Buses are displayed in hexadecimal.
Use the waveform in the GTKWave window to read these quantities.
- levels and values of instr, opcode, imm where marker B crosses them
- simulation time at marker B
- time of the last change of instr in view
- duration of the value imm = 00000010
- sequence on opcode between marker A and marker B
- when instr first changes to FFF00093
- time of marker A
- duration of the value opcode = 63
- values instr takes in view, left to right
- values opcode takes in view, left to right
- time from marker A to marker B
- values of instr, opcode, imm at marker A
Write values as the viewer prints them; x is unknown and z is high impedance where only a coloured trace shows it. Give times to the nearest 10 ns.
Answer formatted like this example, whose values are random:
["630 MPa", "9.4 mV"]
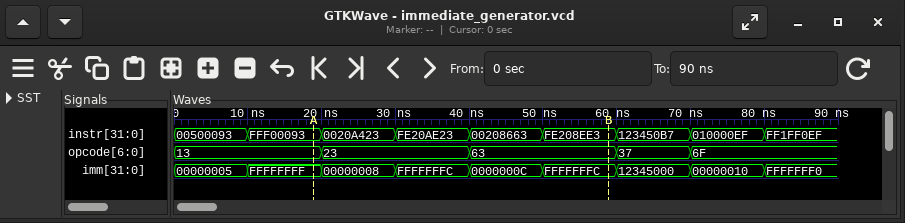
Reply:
["instr=FE208EE3, opcode=63, imm=FFFFFFFC", "60 ns", "80 ns", "10 ns", "13, 23, 63", "10 ns", "20 ns", "20 ns", "00500093, FFF00093, 0020A423, FE20AE23, 00208663, FE208EE3, 123450B7, 010000EF, FF1FF0EF", "13, 23, 63, 37, 6F", "40 ns", "instr=FFF00093, opcode=13, imm=FFFFFFFF"]
